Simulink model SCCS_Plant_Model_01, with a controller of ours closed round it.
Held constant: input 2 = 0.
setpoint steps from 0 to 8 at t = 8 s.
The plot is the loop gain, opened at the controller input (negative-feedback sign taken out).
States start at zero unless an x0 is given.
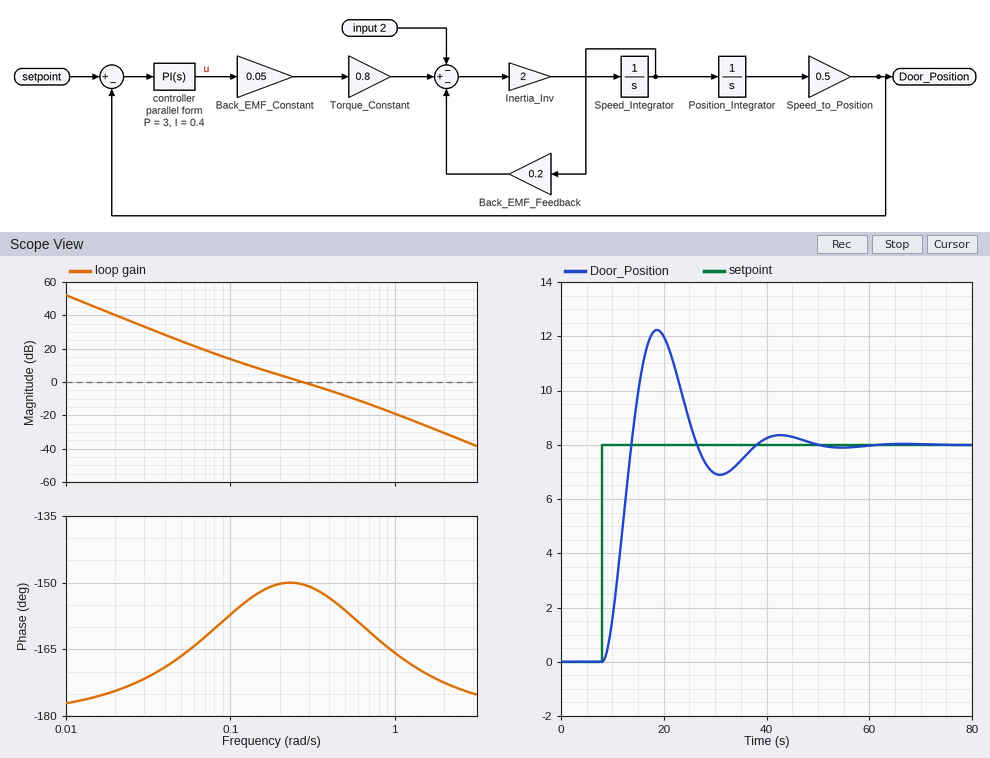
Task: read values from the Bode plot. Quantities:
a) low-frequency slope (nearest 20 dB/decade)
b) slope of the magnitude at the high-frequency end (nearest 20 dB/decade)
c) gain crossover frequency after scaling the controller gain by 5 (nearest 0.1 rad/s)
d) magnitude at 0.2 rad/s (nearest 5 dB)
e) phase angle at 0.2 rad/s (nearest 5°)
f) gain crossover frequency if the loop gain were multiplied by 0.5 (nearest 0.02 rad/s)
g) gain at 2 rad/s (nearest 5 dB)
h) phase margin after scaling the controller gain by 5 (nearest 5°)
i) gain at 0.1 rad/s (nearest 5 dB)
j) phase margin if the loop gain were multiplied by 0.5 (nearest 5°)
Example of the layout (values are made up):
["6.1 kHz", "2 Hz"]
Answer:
["-40 dB/decade", "-40 dB/decade", "0.7 rad/s", "5 dB", "-150°", "0.18 rad/s", "-30 dB", "20°", "15 dB", "30°"]
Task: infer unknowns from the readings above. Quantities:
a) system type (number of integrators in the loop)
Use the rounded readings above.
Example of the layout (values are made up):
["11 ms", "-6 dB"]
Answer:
["2"]
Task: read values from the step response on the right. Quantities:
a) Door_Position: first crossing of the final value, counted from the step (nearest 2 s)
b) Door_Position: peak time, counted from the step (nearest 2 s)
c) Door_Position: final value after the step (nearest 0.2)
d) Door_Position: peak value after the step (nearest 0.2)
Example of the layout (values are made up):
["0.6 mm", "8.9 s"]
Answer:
["6 s", "10 s", "8.0", "12.2"]
